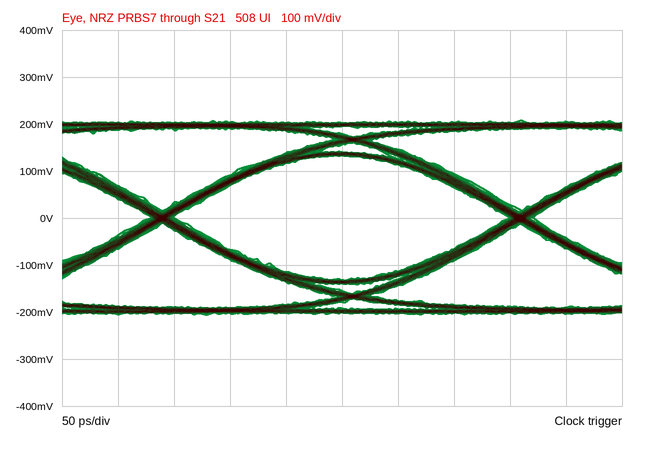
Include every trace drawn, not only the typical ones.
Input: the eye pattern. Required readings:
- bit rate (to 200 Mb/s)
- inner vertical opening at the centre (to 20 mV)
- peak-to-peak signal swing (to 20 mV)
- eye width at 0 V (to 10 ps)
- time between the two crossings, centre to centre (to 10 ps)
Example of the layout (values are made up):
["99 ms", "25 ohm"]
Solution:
["3.2 Gb/s", "260 mV", "420 mV", "300 ps", "320 ps"]
